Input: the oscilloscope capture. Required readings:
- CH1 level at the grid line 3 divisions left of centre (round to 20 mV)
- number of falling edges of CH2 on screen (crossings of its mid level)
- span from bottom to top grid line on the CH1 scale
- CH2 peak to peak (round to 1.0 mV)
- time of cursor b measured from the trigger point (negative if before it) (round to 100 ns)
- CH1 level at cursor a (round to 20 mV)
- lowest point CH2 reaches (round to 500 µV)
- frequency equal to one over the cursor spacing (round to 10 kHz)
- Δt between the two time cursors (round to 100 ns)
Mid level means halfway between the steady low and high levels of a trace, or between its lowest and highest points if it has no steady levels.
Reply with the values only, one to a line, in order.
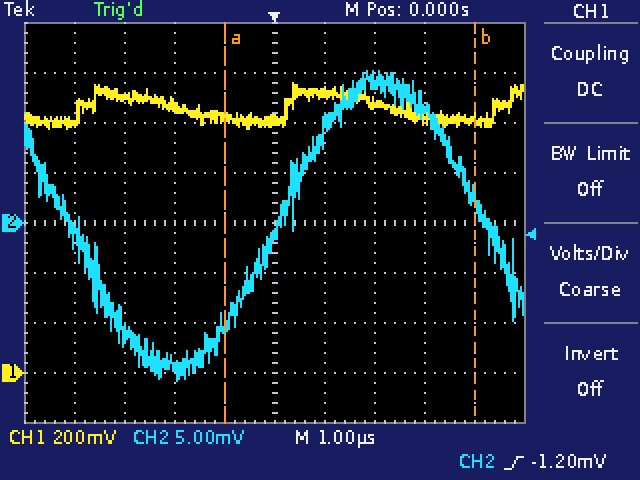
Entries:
1.10 V
2
1.6 V
31.0 mV
+4.0 µs
1.02 V
-16.0 mV
200 kHz
5.0 µs
